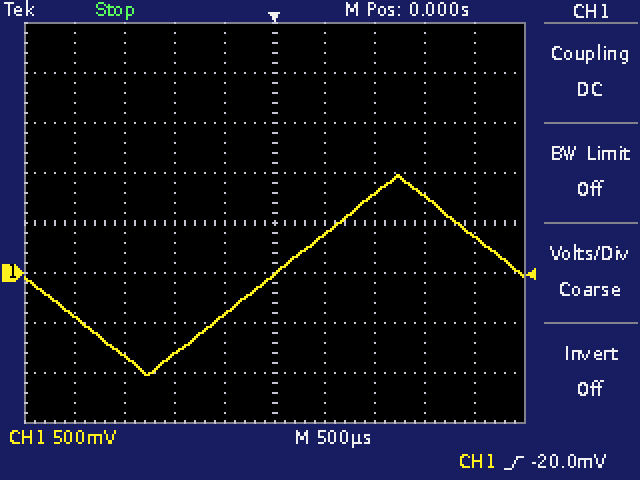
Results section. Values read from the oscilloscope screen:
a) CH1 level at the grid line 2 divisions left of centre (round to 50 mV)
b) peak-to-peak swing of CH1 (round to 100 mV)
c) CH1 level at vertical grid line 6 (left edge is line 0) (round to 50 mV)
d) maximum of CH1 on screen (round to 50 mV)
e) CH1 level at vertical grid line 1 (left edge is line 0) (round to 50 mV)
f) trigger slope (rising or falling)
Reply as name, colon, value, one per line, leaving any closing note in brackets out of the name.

CH1 level at the grid line 2 divisions left of centre: -800 mV
peak-to-peak swing of CH1: 2.00 V
CH1 level at vertical grid line 6 (left edge is line 0): 400 mV
maximum of CH1 on screen: 1.00 V
CH1 level at vertical grid line 1 (left edge is line 0): -450 mV
trigger slope: rising
